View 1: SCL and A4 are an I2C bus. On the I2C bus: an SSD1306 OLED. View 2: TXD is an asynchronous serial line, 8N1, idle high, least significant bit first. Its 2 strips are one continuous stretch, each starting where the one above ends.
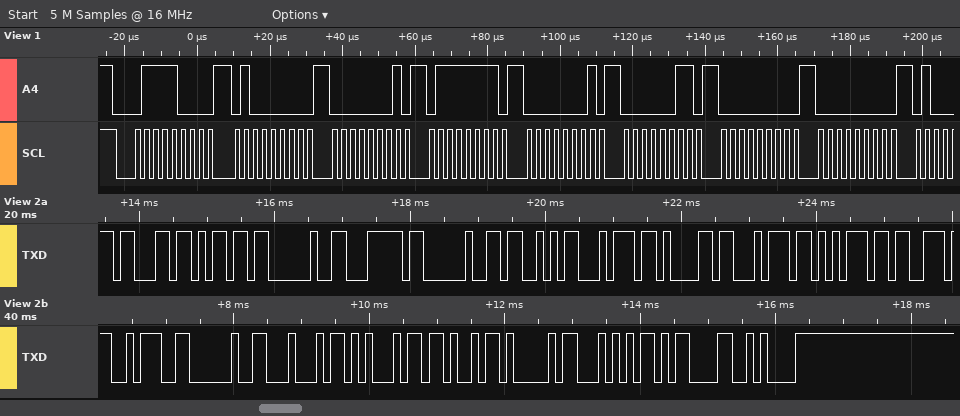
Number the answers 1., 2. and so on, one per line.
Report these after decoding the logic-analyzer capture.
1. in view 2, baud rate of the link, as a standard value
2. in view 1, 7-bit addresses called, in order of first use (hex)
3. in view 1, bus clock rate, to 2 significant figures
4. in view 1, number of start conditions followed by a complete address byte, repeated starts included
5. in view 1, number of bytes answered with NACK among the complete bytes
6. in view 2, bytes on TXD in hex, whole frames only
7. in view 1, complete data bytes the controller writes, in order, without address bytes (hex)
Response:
1. 9600 baud
2. 0x3C
3. 400 kHz
4. 1
5. 0
6. 63 6D 20 7C 20 53 74 61 74 75 73 3A 20 44 45 4B 41 54 0D 0A
7. 40 01 7F 01 03 00 00
